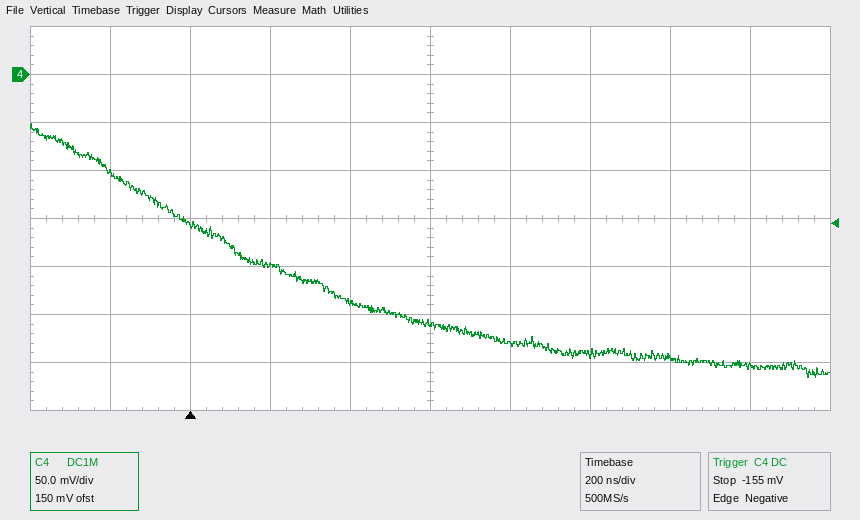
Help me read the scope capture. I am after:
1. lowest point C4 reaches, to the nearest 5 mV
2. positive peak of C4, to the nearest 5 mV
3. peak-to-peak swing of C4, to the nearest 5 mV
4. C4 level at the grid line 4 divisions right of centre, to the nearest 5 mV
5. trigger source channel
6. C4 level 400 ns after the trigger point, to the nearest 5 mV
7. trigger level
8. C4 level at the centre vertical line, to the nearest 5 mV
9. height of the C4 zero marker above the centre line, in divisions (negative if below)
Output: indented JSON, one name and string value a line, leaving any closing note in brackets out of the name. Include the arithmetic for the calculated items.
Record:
{
  "lowest point C4 reaches, to the nearest 5 mV": "-315 mV",
  "positive peak of C4, to the nearest 5 mV": "-50 mV",
  "peak-to-peak swing of C4, to the nearest 5 mV": "-50 mV − (-315 mV) = 265 mV",
  "C4 level at the grid line 4 divisions right of centre, to the nearest 5 mV": "-305 mV",
  "trigger source channel": "C4",
  "C4 level 400 ns after the trigger point, to the nearest 5 mV": "-235 mV",
  "trigger level": "-155 mV",
  "C4 level at the centre vertical line, to the nearest 5 mV": "-260 mV",
  "height of the C4 zero marker above the centre line, in divisions": "+3.0 div"
}
